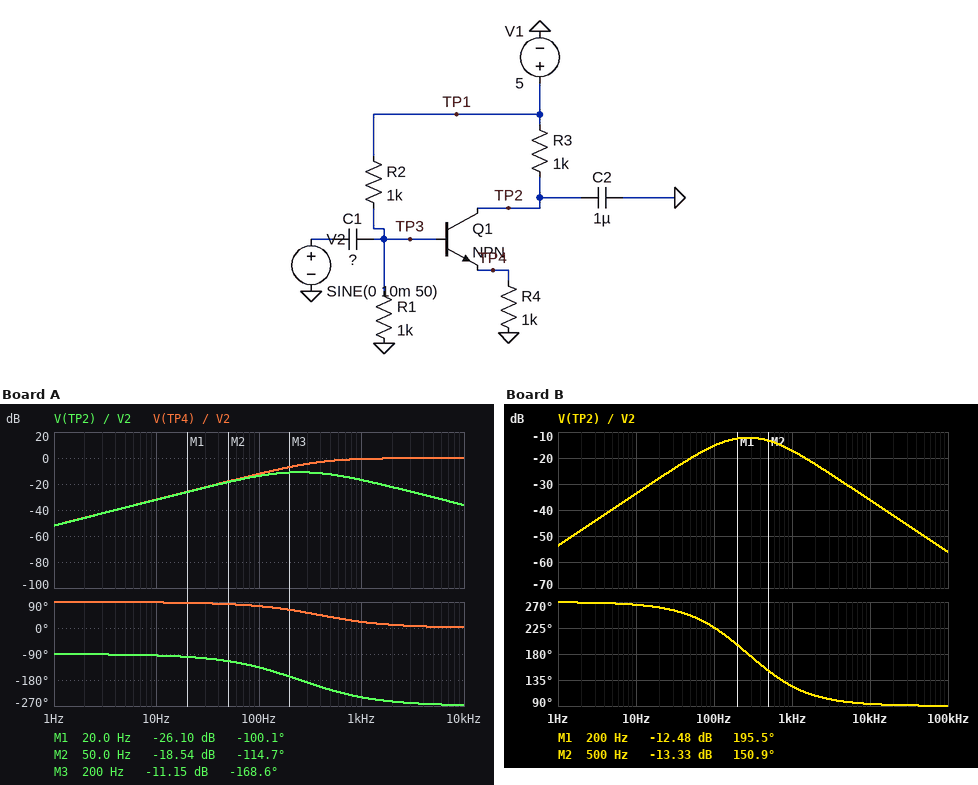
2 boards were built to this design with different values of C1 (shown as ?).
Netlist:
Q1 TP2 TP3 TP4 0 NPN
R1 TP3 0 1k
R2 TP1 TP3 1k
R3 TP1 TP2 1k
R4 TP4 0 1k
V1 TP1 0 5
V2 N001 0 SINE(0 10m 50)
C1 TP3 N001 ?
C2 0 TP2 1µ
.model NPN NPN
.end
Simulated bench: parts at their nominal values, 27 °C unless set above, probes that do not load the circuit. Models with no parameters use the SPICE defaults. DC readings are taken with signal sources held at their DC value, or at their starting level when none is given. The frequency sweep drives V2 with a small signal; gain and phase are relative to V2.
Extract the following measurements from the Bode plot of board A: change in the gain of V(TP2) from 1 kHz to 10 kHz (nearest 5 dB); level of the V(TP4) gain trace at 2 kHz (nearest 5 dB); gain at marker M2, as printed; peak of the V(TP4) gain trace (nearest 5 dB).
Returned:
-20 dB
0 dB
-18.54 dB
0 dB
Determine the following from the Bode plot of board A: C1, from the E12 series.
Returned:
820 nF
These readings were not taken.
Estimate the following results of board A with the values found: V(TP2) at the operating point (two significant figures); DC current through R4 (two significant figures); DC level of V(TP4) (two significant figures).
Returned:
3.3 V
1.7 mA
1.7 V
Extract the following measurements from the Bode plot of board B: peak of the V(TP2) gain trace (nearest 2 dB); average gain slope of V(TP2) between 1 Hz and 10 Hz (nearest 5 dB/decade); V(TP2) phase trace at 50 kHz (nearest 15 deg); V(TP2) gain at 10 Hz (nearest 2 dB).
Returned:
-12 dB
20 dB/decade
90 deg
-34 dB
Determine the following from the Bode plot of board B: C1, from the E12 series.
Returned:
680 nF
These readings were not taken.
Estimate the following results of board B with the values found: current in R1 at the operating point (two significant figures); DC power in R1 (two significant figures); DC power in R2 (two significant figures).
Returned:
2.5 mA
6.2 mW
6.3 mW
